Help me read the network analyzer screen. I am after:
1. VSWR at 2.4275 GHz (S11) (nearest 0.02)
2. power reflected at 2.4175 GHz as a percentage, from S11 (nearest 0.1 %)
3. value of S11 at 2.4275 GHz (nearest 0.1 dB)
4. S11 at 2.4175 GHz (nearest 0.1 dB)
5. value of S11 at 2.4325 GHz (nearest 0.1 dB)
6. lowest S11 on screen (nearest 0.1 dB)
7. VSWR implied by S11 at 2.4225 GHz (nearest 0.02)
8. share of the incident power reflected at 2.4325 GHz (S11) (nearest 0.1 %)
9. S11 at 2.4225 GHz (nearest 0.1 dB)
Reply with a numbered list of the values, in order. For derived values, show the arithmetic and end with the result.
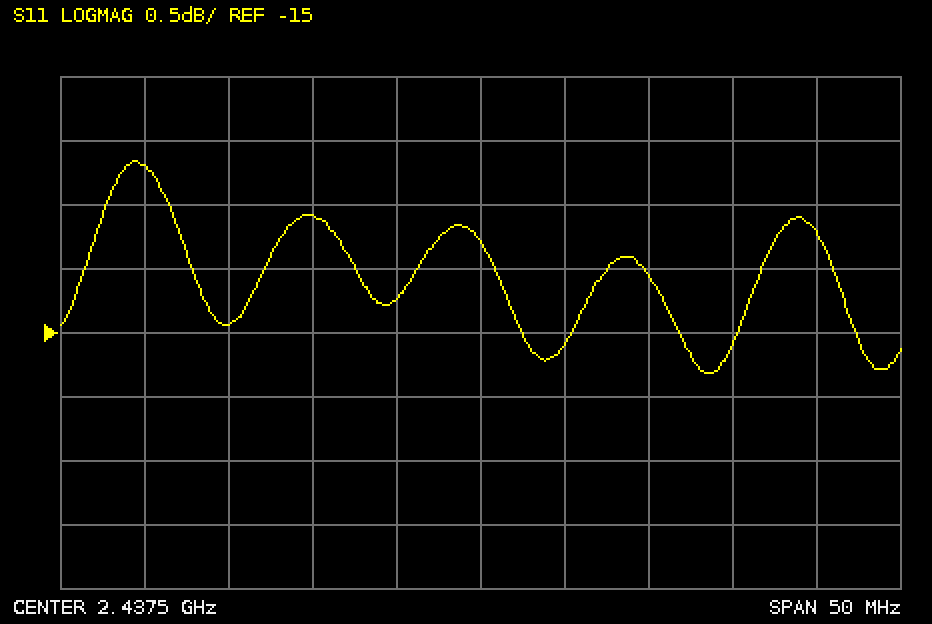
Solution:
1. |Γ| = 10^(-14.1/20) = 0.1972; VSWR = (1 + 0.1972)/(1 − 0.1972) ≈ 1.49, so 1.50 to the nearest 0.02
2. 10^(-13.7/10) ≈ 4.3 %
3. -14.1 dB
4. -13.7 dB
5. -14.7 dB
6. -15.3 dB
7. |Γ| = 10^(-14.9/20) = 0.1799; VSWR = (1 + 0.1799)/(1 − 0.1799) ≈ 1.44
8. 10^(-14.7/10) ≈ 3.4 %
9. -14.9 dB
